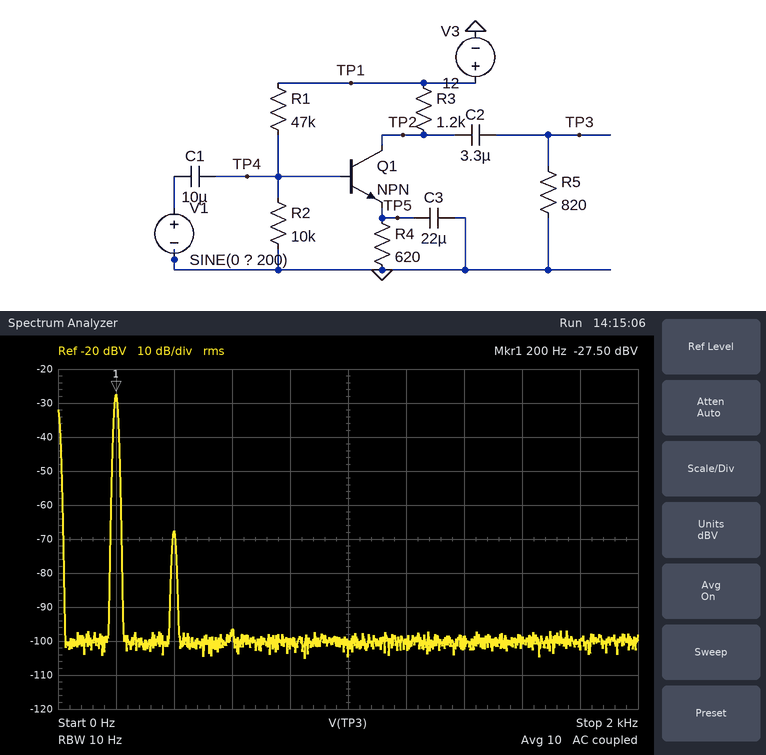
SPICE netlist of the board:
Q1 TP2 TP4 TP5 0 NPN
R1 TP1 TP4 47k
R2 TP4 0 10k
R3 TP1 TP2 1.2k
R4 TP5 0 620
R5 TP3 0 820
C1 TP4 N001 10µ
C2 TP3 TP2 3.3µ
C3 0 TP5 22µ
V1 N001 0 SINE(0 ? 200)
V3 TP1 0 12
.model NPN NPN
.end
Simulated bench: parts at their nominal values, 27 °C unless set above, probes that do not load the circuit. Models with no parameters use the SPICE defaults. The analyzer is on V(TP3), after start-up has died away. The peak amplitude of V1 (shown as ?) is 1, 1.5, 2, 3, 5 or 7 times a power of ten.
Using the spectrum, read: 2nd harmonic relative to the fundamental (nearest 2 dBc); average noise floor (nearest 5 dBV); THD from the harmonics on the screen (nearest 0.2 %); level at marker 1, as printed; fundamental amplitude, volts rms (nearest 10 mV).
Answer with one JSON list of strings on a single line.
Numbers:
["-40 dBc", "-100 dBV", "1.0 %", "-27.50 dBV", "40 mV"]
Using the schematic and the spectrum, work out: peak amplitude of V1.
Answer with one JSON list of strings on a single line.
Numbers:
["5 mV"]
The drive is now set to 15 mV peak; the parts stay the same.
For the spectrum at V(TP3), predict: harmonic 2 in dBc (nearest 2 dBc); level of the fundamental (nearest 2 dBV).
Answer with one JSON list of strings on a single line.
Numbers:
["-30 dBc", "-18 dBV"]
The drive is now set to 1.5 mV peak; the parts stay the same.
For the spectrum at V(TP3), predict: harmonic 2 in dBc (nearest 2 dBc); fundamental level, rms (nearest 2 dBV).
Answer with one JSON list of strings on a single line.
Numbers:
["-50 dBc", "-38 dBV"]
